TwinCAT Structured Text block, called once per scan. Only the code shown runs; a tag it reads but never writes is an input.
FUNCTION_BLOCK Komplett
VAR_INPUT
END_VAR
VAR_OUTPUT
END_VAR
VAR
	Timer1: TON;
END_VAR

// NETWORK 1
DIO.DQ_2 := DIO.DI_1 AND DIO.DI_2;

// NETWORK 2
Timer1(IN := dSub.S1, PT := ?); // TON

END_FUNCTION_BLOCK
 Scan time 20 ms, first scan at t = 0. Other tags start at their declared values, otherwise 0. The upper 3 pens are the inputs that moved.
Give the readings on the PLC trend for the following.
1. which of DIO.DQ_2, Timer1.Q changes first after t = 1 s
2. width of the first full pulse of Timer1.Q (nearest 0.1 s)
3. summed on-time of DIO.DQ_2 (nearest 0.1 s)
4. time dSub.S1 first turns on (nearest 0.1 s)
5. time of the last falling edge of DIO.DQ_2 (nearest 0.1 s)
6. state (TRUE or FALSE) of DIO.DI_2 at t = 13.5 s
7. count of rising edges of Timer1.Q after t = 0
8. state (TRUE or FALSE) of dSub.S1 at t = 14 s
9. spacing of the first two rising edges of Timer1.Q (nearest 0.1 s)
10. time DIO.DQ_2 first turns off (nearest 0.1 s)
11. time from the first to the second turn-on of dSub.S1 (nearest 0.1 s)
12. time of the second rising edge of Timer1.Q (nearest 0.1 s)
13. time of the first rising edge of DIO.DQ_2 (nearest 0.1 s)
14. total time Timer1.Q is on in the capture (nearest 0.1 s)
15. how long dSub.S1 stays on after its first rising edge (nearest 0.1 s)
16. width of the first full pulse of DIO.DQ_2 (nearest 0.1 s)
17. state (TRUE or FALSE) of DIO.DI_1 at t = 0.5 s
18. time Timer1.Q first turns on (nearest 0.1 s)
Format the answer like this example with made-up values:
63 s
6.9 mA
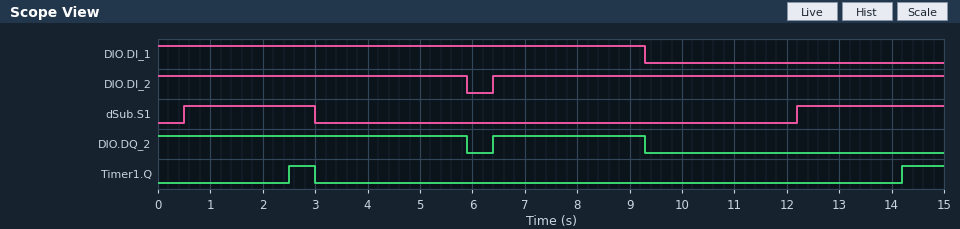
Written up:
Timer1.Q
0.5 s
8.8 s
0.5 s
9.3 s
TRUE
2
TRUE
11.7 s
5.9 s
11.7 s
14.2 s
6.4 s
1.3 s
2.5 s
2.9 s
TRUE
2.5 s
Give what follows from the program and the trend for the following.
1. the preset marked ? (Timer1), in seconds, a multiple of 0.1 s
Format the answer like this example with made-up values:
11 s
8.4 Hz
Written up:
2.0 s
